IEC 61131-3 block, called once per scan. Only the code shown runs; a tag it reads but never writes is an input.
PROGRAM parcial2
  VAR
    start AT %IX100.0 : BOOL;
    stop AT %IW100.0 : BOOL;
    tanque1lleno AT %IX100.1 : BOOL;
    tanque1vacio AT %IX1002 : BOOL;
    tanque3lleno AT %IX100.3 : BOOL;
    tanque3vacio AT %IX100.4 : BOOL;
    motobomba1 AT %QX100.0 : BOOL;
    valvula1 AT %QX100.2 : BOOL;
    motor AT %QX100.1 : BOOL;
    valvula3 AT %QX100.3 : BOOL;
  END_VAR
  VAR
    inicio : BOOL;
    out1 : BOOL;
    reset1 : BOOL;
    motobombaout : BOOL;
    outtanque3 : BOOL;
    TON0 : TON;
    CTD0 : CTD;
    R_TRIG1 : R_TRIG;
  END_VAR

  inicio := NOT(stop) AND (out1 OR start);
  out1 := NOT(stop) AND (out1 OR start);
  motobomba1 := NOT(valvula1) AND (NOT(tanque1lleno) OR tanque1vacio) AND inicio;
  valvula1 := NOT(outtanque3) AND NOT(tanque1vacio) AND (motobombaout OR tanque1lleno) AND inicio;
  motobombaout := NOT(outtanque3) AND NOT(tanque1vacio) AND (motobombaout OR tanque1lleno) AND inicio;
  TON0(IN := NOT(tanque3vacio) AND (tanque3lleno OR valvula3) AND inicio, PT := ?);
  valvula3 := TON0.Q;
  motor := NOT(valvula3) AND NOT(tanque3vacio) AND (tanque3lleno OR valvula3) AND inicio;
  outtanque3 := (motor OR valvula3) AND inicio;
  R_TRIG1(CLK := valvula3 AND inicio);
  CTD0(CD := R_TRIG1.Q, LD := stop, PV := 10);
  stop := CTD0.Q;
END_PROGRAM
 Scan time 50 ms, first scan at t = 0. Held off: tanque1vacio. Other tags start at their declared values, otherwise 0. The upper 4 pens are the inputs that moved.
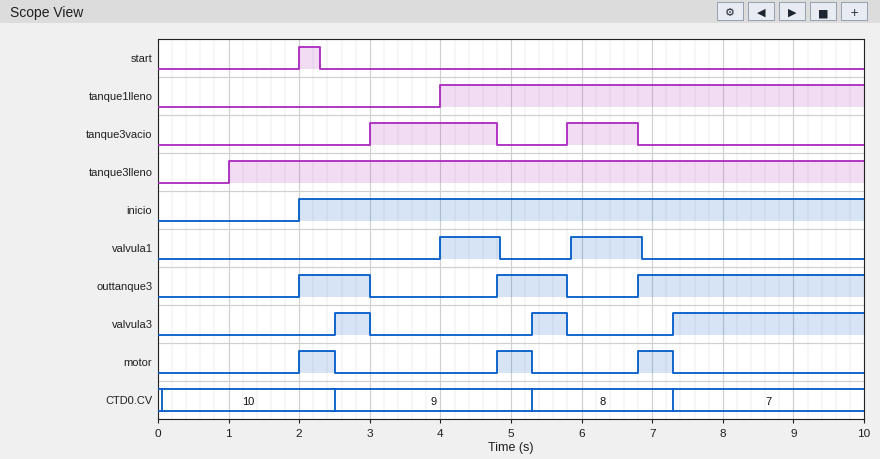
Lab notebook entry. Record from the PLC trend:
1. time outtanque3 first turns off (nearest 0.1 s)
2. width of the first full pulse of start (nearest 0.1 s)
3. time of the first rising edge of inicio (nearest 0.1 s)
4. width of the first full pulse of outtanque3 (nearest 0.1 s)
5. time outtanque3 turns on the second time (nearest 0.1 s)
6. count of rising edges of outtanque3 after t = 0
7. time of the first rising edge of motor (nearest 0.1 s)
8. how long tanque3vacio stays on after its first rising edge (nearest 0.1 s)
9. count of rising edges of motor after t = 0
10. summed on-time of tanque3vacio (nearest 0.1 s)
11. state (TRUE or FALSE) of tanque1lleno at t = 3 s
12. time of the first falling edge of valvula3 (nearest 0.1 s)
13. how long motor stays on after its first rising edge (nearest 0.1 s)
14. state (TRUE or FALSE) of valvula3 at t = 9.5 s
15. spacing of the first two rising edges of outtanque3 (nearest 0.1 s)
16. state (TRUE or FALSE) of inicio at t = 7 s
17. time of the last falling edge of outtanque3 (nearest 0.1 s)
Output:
3.0 s
0.3 s
2.0 s
1.0 s
4.8 s
3
2.0 s
1.8 s
3
2.8 s
FALSE
3.0 s
0.5 s
TRUE
2.8 s
TRUE
5.8 s
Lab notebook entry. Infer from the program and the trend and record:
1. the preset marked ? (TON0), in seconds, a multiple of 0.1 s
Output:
0.5 s
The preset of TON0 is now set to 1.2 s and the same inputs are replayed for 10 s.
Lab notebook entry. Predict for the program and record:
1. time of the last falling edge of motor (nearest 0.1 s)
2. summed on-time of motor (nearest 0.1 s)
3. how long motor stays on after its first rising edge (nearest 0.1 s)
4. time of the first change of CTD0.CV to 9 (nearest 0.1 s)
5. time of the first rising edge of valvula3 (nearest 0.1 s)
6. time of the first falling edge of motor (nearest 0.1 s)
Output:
8.0 s
3.2 s
1.0 s
8.0 s
8.0 s
3.0 s
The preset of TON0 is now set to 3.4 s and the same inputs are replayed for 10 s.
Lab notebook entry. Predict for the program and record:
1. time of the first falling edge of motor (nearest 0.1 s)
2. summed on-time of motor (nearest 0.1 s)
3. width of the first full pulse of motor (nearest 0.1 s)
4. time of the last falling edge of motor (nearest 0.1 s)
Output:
3.0 s
5.2 s
1.0 s
5.8 s
